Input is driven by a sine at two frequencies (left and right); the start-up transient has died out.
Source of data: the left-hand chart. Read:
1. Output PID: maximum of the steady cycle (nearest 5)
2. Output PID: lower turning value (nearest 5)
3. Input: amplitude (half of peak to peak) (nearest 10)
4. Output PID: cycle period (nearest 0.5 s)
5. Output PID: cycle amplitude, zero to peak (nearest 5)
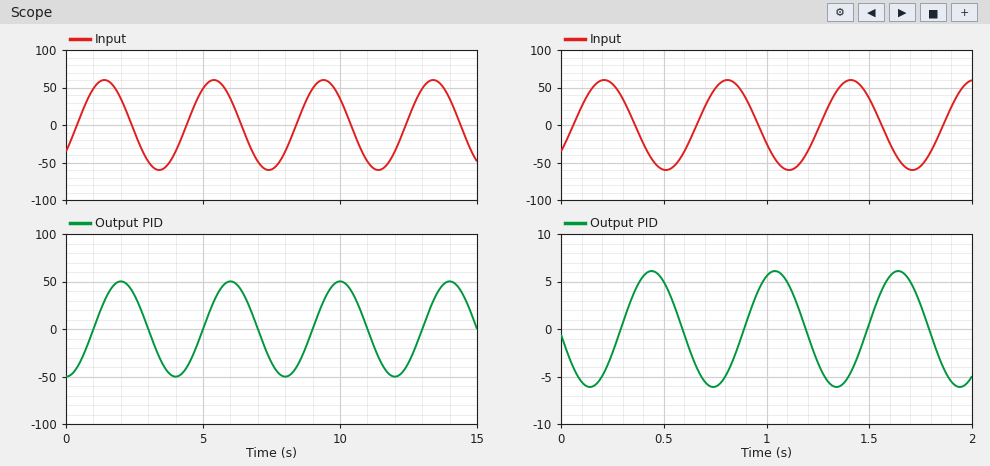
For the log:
50
-50
60
4.0 s
50
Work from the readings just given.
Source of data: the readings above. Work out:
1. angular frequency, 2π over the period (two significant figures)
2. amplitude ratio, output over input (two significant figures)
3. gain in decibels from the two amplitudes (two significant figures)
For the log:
1.6 rad/s
0.83
-1.6 dB
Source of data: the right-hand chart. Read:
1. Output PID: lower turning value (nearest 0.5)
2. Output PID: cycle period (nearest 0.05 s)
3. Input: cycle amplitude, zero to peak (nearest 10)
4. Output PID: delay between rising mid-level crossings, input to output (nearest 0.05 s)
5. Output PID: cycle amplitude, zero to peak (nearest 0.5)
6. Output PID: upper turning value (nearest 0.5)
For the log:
-6.0
0.60 s
60
0.25 s
6.0
6.0
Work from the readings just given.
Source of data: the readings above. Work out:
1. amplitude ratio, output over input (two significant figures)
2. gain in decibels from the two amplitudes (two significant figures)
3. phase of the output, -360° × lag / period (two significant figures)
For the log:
0.10
-20 dB
-150°
